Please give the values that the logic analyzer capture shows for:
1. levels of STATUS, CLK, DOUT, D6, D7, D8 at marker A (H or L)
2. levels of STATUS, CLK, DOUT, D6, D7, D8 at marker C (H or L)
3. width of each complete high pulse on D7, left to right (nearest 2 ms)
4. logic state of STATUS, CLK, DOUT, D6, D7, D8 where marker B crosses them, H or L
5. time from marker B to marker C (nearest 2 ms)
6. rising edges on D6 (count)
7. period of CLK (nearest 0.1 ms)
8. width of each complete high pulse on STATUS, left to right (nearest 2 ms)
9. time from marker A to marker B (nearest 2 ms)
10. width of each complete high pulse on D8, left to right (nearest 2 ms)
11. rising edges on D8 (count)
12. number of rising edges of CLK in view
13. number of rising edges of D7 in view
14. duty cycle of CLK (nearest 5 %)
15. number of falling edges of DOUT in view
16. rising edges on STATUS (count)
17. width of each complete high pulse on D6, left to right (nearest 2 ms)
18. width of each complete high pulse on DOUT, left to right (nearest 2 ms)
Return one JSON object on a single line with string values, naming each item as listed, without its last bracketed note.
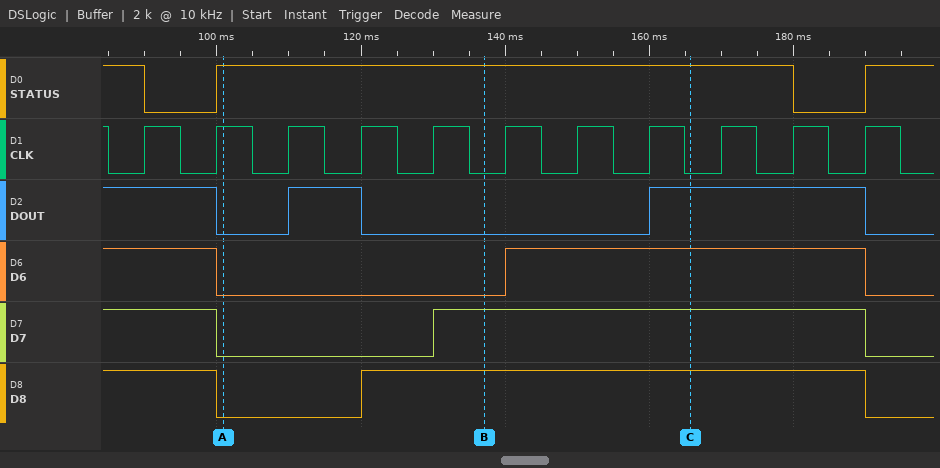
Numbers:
{"levels of STATUS, CLK, DOUT, D6, D7, D8 at marker A": "STATUS=H, CLK=H, DOUT=L, D6=L, D7=L, D8=L", "levels of STATUS, CLK, DOUT, D6, D7, D8 at marker C": "STATUS=H, CLK=L, DOUT=H, D6=H, D7=H, D8=H", "width of each complete high pulse on D7, left to right": "60 ms", "logic state of STATUS, CLK, DOUT, D6, D7, D8 where marker B crosses them, H or L": "STATUS=H, CLK=L, DOUT=L, D6=L, D7=H, D8=H", "time from marker B to marker C": "28 ms", "rising edges on D6": "1", "period of CLK": "10 ms", "width of each complete high pulse on STATUS, left to right": "80 ms", "time from marker A to marker B": "36 ms", "width of each complete high pulse on D8, left to right": "70 ms", "rising edges on D8": "1", "number of rising edges of CLK in view": "11", "number of rising edges of D7 in view": "1", "duty cycle of CLK": "50 %", "number of falling edges of DOUT in view": "3", "rising edges on STATUS": "2", "width of each complete high pulse on D6, left to right": "50 ms", "width of each complete high pulse on DOUT, left to right": "10 ms, 30 ms"}
